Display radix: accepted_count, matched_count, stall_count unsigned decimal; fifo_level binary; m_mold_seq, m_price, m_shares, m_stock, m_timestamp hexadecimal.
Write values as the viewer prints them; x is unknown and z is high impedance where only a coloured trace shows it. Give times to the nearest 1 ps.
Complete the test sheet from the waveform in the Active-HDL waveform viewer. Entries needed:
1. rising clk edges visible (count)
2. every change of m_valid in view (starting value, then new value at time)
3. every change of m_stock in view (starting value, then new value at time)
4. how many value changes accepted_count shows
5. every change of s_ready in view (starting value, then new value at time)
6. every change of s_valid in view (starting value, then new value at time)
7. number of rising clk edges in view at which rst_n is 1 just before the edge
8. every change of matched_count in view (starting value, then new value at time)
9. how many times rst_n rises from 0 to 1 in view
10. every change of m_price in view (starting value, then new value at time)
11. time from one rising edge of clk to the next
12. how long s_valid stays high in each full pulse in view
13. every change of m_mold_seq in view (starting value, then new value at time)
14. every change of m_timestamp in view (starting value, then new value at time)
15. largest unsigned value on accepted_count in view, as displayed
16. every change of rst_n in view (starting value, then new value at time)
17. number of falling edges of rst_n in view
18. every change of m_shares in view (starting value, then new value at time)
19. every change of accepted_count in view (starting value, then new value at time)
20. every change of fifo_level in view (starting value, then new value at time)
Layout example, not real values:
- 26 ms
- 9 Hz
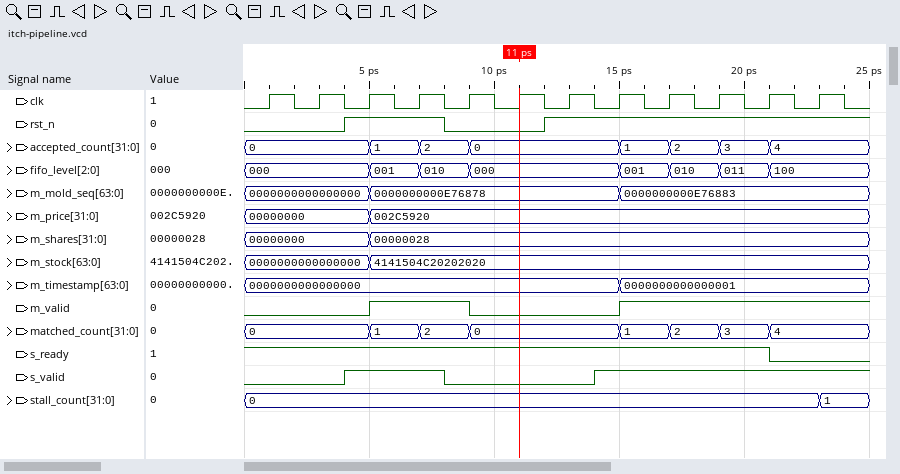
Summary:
- 12
- 0, 1 at 5 ps, 0 at 9 ps, 1 at 15 ps
- 0000000000000000, 4141504C20202020 at 5 ps
- 7
- 1, 0 at 21 ps
- 0, 1 at 4 ps, 0 at 8 ps, 1 at 14 ps
- 8
- 0, 1 at 5 ps, 2 at 7 ps, 0 at 9 ps, 1 at 15 ps, 2 at 17 ps, 3 at 19 ps, 4 at 21 ps
- 2
- 00000000, 002C5920 at 5 ps
- 2 ps
- 4 ps
- 0000000000000000, 0000000000E76878 at 5 ps, 0000000000E76883 at 15 ps
- 0000000000000000, 0000000000000001 at 15 ps
- 4
- 0, 1 at 4 ps, 0 at 8 ps, 1 at 12 ps
- 1
- 00000000, 00000028 at 5 ps
- 0, 1 at 5 ps, 2 at 7 ps, 0 at 9 ps, 1 at 15 ps, 2 at 17 ps, 3 at 19 ps, 4 at 21 ps
- 000, 001 at 5 ps, 010 at 7 ps, 000 at 9 ps, 001 at 15 ps, 010 at 17 ps, 011 at 19 ps, 100 at 21 ps
